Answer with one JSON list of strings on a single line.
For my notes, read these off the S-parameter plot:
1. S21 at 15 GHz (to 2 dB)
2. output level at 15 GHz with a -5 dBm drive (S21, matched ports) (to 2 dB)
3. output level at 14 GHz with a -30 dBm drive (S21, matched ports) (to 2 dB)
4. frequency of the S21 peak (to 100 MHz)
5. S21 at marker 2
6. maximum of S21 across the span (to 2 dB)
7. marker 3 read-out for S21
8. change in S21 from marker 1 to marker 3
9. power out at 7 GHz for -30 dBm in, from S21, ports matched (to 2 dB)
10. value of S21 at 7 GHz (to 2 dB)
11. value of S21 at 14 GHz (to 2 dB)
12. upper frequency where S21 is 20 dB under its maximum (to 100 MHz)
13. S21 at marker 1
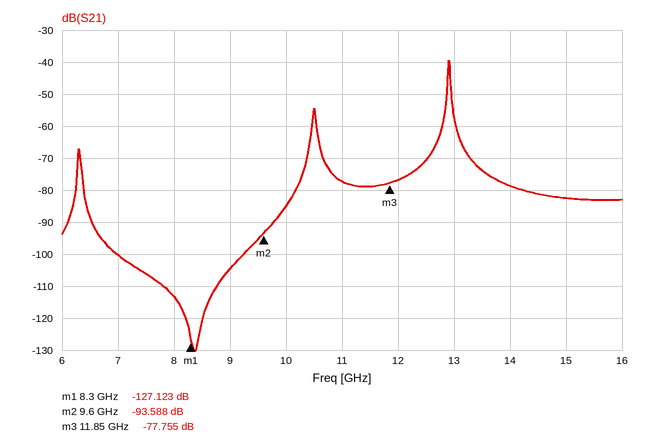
["-82 dB", "-88 dBm", "-108 dBm", "12.9 GHz", "-93.588 dB", "-40 dB", "-77.755 dB", "49.368 dB", "-130 dBm", "-100 dB", "-78 dB", "13.0 GHz", "-127.123 dB"]
